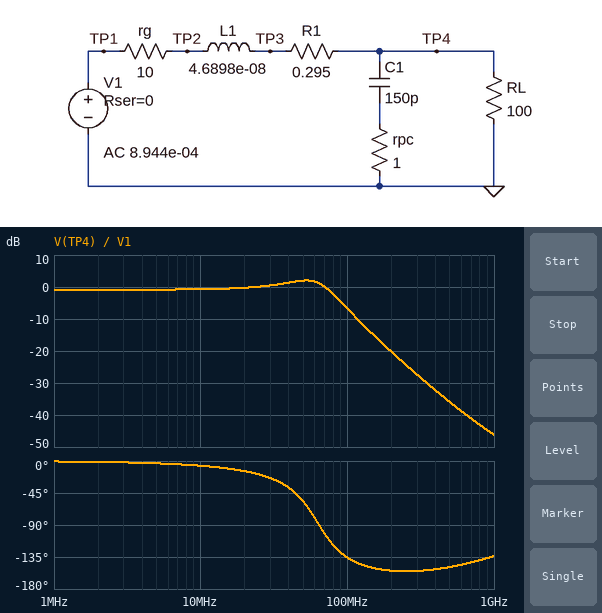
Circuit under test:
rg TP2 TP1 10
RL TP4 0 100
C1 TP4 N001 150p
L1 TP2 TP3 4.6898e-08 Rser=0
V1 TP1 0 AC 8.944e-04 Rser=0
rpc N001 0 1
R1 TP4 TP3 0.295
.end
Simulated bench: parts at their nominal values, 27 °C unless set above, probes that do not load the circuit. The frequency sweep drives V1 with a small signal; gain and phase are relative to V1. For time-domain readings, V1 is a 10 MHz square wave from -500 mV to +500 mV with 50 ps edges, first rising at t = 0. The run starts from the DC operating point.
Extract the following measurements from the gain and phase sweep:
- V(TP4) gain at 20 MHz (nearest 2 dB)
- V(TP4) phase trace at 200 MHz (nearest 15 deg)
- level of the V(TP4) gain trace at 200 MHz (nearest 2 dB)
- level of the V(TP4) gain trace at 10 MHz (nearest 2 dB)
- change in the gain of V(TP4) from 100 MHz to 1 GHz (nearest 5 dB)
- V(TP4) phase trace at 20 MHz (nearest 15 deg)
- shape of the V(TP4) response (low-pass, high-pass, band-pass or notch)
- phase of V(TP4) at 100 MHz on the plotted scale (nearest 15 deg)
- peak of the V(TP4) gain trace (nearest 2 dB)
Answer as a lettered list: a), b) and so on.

a) 0 dB
b) -150 deg
c) -20 dB
d) 0 dB
e) -40 dB
f) -15 deg
g) low-pass
h) -135 deg
i) 2 dB
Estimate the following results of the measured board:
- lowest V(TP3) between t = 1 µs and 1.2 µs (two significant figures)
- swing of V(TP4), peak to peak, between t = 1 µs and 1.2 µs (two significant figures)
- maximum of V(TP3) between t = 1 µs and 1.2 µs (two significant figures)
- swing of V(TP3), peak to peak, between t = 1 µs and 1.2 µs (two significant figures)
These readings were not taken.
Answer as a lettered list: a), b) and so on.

a) -700 mV
b) 1.4 V
c) 700 mV
d) 1.4 V
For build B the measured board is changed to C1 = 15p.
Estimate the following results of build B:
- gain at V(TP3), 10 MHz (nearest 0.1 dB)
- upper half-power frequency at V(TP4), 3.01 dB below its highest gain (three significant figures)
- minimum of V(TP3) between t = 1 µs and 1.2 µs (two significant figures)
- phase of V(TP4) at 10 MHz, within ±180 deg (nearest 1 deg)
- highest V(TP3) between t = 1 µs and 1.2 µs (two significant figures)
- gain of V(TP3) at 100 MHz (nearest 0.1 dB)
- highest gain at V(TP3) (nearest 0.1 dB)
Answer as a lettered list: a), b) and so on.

a) -0.8 dB
b) 236 MHz
c) -730 mV
d) -2 deg
e) 730 mV
f) 0.8 dB
g) 2.6 dB
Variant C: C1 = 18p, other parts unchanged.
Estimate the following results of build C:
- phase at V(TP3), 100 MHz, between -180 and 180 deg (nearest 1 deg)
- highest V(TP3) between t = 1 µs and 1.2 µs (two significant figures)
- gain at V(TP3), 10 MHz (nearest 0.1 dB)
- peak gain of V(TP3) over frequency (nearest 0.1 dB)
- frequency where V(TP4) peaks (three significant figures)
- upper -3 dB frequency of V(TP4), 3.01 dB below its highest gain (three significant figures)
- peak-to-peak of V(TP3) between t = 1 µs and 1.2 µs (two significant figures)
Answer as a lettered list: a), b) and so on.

a) -28 deg
b) 740 mV
c) -0.8 dB
d) 2.9 dB
e) 158 MHz
f) 215 MHz
g) 1.5 V
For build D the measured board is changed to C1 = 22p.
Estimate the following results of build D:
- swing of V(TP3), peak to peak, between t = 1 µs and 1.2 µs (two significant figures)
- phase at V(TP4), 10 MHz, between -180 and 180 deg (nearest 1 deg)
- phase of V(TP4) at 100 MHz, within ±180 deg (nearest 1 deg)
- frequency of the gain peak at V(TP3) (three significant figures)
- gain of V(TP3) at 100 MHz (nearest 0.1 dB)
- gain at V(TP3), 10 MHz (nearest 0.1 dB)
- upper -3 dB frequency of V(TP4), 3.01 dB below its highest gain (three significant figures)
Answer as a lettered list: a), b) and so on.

a) 1.5 V
b) -2 deg
c) -32 deg
d) 144 MHz
e) 1.7 dB
f) -0.8 dB
g) 194 MHz
